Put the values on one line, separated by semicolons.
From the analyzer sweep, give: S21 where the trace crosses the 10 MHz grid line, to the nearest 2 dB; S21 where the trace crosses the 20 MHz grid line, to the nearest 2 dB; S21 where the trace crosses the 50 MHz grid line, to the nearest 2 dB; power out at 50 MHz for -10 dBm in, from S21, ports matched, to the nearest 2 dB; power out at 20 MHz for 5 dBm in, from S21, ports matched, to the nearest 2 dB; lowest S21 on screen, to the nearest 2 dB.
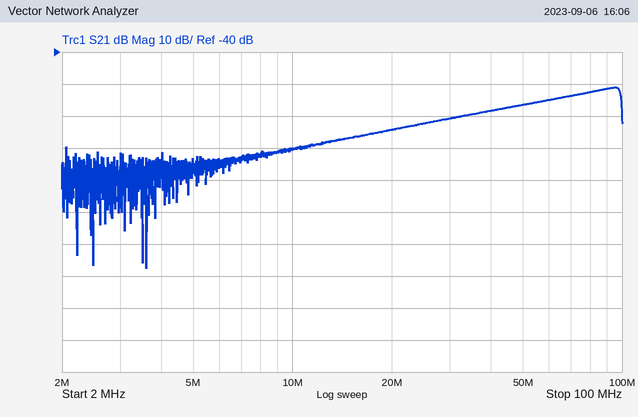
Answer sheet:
-70 dB; -64 dB; -56 dB; -66 dBm; -60 dBm; -108 dB
